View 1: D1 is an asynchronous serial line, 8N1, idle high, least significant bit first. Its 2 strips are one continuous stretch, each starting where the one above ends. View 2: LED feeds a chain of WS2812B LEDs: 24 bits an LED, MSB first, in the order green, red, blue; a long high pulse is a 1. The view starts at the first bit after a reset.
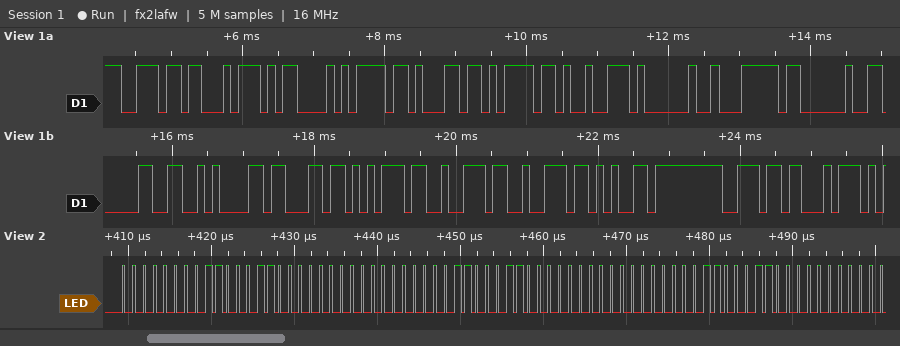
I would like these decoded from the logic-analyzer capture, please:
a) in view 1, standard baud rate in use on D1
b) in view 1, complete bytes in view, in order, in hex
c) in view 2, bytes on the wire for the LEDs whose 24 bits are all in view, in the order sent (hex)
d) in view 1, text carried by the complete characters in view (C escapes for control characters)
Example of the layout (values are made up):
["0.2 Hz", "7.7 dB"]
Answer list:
["9600 baud", "6E 74 43 6F 6C 6F 72 20 7C 20 30 0A 63 75 72 72 65 6E 74", "00 C6 00 00 C6 00 00 C6 00", "\"ntColor | 0\\ncurrent\""]
